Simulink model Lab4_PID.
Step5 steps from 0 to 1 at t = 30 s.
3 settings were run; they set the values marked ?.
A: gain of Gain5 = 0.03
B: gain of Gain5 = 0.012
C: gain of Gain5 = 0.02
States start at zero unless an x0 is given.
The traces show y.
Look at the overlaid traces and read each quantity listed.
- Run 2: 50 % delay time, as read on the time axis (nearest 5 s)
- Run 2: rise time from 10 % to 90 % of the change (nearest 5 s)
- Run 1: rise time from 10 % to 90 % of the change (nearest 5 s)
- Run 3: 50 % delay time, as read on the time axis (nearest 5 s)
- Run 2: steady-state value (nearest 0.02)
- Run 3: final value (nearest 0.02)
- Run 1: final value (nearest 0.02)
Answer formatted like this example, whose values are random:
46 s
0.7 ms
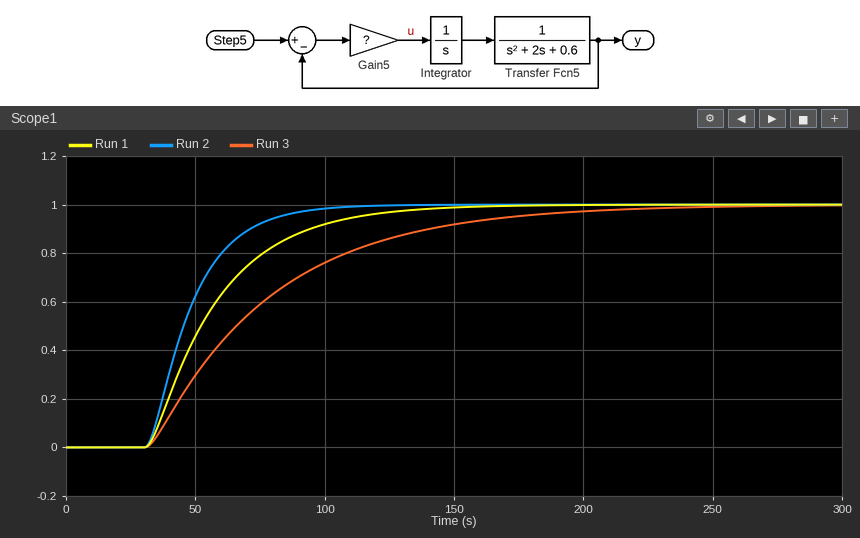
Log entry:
45 s
35 s
60 s
65 s
1.00
1.00
1.00
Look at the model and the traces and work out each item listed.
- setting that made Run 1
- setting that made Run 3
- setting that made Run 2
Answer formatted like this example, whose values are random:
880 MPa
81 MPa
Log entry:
C
B
A
